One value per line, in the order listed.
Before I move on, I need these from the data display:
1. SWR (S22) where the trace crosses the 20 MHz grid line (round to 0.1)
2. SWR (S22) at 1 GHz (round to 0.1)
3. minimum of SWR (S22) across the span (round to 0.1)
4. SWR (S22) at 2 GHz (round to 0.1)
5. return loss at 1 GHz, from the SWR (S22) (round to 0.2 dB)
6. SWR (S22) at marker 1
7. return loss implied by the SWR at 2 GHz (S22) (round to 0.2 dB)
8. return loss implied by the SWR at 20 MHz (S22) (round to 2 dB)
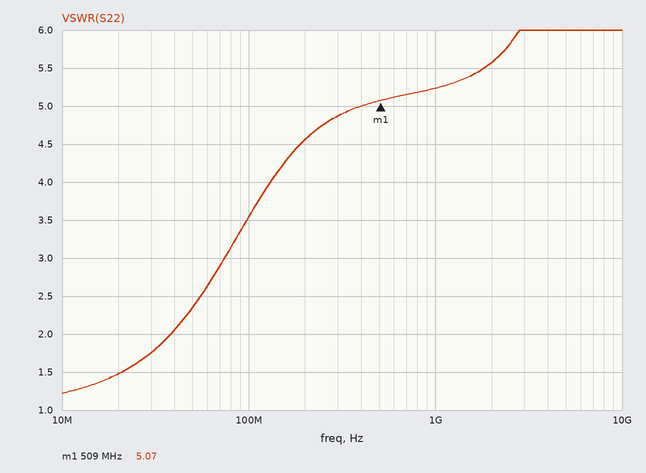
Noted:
1.5
5.2
1.2
5.6
3.4 dB
5.07
3.2 dB
14 dB
